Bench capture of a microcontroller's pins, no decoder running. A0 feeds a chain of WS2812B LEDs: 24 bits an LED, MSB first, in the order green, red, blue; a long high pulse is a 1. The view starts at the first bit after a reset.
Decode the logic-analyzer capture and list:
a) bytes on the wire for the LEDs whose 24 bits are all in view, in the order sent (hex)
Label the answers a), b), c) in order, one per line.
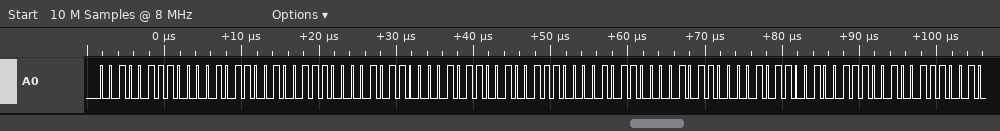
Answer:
a) 27 0B 27 0B 0B 27 0B 0B 0B
